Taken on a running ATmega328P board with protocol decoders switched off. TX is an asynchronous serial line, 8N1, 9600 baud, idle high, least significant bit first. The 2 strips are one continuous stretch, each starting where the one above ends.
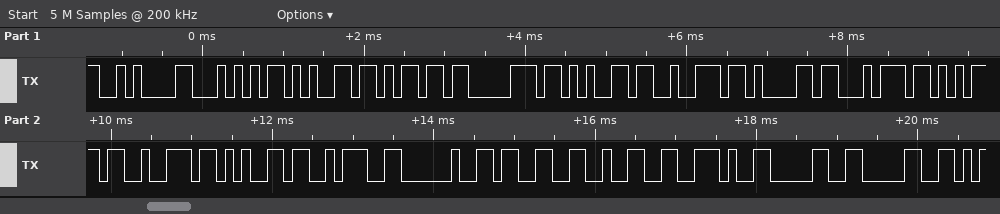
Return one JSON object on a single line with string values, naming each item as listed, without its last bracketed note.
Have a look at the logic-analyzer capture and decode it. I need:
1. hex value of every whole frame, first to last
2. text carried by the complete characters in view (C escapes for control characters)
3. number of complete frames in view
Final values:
{"hex value of every whole frame, first to last": "0x0A 0x54 0x65 0x6D 0x70 0x65 0x72 0x61 0x74 0x75 0x72 0x65 0x3A 0x20 0x33 0x32 0x2E 0x30 0x30", "text carried by the complete characters in view": "\"\\nTemperature: 32.00\"", "number of complete frames in view": "19"}
